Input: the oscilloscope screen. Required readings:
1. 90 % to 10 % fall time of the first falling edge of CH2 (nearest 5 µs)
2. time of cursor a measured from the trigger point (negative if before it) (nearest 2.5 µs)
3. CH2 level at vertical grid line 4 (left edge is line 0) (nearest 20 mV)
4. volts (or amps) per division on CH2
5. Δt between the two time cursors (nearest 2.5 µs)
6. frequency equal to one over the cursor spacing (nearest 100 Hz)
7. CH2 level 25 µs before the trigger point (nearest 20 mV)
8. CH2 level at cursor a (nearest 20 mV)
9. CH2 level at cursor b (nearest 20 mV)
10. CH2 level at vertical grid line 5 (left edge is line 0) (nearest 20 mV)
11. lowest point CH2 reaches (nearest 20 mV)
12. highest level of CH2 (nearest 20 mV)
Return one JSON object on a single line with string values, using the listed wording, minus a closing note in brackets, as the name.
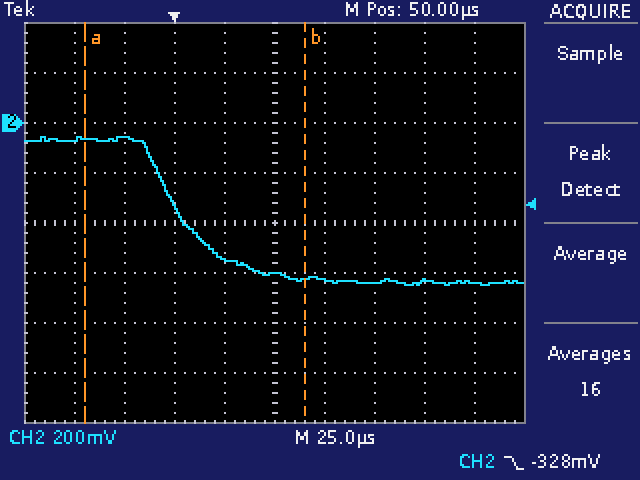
{"90 % to 10 % fall time of the first falling edge of CH2": "50 µs", "time of cursor a measured from the trigger point (negative if before it)": "-45.0 µs", "CH2 level at vertical grid line 4 (left edge is line 0)": "-540 mV", "volts (or amps) per division on CH2": "200 mV", "Δt between the two time cursors": "110.0 µs", "frequency equal to one over the cursor spacing": "9.1 kHz", "CH2 level 25 µs before the trigger point": "-60 mV", "CH2 level at cursor a": "-60 mV", "CH2 level at cursor b": "-620 mV", "CH2 level at vertical grid line 5 (left edge is line 0)": "-600 mV", "lowest point CH2 reaches": "-640 mV", "highest level of CH2": "-60 mV"}
